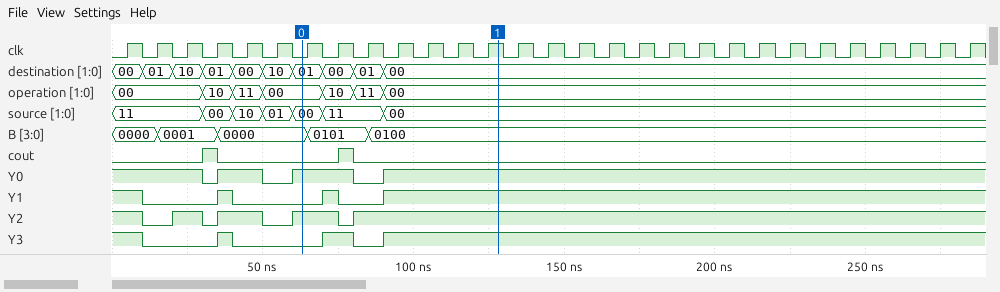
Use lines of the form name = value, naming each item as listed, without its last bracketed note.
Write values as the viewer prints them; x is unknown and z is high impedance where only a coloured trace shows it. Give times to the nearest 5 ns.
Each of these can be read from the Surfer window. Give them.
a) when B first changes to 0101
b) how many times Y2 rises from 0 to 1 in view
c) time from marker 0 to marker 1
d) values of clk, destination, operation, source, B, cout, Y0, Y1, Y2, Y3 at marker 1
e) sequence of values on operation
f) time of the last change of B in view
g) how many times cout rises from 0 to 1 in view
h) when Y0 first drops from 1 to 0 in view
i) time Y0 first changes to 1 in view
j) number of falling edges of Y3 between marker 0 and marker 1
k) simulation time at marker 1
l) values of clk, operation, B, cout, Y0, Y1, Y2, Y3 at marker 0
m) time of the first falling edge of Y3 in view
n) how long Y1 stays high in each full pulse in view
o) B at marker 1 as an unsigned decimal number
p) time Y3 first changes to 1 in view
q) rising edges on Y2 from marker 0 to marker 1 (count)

when B first changes to 0101 = 65 ns
how many times Y2 rises from 0 to 1 in view = 4
time from marker 0 to marker 1 = 65 ns
values of clk, destination, operation, source, B, cout, Y0, Y1, Y2, Y3 at marker 1 = clk=1, destination=00, operation=00, source=00, B=0100, cout=0, Y0=1, Y1=1, Y2=1, Y3=1
sequence of values on operation = 00, 10, 11, 00, 10, 11, 00
time of the last change of B in view = 85 ns
how many times cout rises from 0 to 1 in view = 2
when Y0 first drops from 1 to 0 in view = 30 ns
time Y0 first changes to 1 in view = 35 ns
number of falling edges of Y3 between marker 0 and marker 1 = 1
simulation time at marker 1 = 130 ns
values of clk, operation, B, cout, Y0, Y1, Y2, Y3 at marker 0 = clk=0, operation=00, B=0000, cout=0, Y0=1, Y1=0, Y2=1, Y3=0
time of the first falling edge of Y3 in view = 10 ns
how long Y1 stays high in each full pulse in view = 5 ns, 5 ns
B at marker 1 as an unsigned decimal number = 4
time Y3 first changes to 1 in view = 35 ns
rising edges on Y2 from marker 0 to marker 1 = 1
